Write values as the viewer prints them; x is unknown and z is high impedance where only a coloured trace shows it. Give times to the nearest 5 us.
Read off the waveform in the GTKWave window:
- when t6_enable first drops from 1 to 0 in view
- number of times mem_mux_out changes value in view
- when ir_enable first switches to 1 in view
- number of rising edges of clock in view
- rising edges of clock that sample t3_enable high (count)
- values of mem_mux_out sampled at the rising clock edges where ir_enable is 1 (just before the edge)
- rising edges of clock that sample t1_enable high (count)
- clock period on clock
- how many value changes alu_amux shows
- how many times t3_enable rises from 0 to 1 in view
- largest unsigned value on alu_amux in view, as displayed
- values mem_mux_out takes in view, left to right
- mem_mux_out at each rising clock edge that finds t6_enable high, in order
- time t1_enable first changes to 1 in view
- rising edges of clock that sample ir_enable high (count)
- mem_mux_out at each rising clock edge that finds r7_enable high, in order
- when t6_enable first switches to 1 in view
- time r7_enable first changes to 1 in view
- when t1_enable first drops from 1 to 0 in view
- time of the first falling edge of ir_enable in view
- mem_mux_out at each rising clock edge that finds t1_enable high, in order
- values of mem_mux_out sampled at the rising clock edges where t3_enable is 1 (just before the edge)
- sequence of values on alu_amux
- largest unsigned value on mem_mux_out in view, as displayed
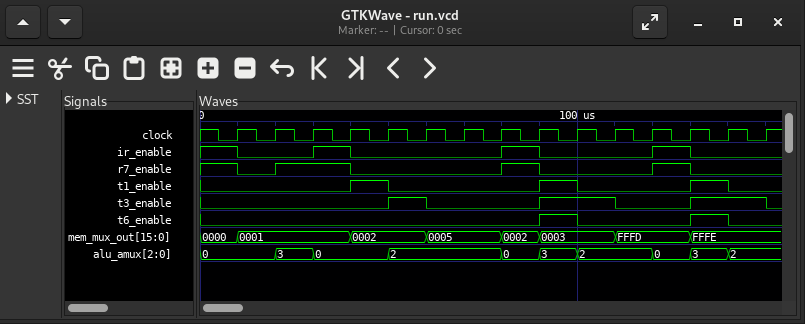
100 us
7
30 us
15
5
0000, 0001, 0002, FFFD
3
10 us
9
3
3
0000, 0001, 0002, 0005, 0002, 0003, FFFD, FFFE
0003, FFFE
40 us
4
0000, 0001, 0001, 0002, FFFD
90 us
20 us
50 us
10 us
0002, 0003, FFFE
0002, 0003, 0003, FFFE, FFFE
0, 3, 0, 2, 0, 3, 2, 0, 3, 2
FFFE
